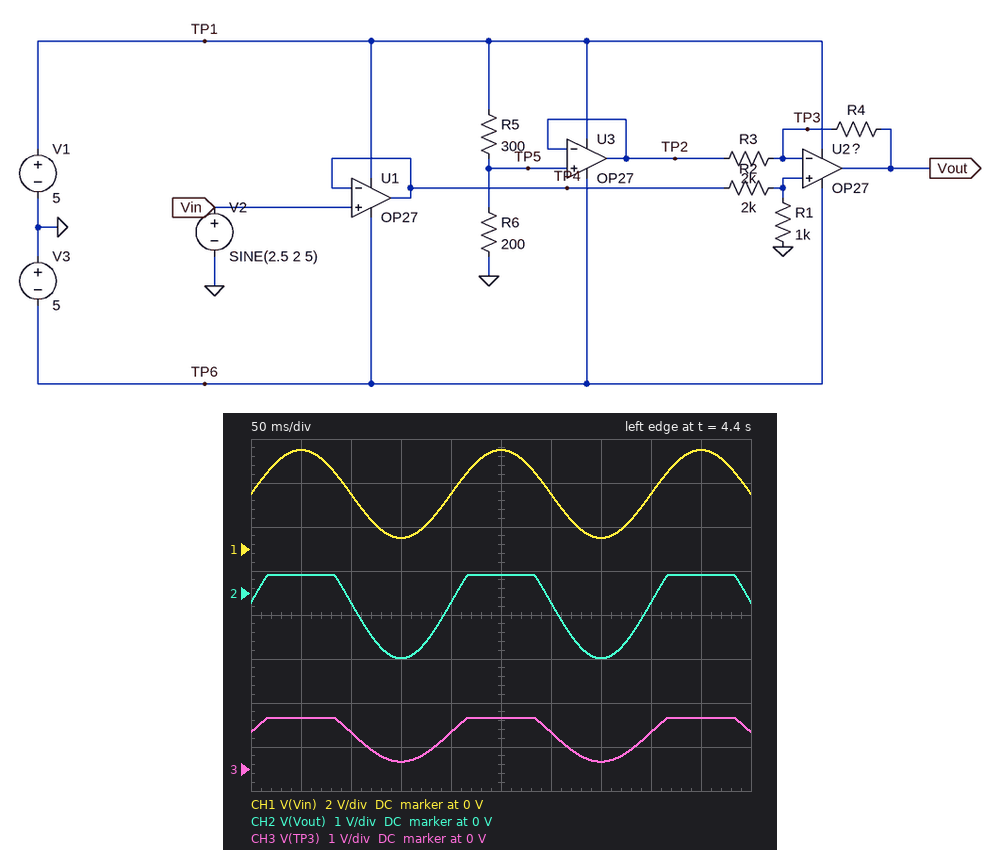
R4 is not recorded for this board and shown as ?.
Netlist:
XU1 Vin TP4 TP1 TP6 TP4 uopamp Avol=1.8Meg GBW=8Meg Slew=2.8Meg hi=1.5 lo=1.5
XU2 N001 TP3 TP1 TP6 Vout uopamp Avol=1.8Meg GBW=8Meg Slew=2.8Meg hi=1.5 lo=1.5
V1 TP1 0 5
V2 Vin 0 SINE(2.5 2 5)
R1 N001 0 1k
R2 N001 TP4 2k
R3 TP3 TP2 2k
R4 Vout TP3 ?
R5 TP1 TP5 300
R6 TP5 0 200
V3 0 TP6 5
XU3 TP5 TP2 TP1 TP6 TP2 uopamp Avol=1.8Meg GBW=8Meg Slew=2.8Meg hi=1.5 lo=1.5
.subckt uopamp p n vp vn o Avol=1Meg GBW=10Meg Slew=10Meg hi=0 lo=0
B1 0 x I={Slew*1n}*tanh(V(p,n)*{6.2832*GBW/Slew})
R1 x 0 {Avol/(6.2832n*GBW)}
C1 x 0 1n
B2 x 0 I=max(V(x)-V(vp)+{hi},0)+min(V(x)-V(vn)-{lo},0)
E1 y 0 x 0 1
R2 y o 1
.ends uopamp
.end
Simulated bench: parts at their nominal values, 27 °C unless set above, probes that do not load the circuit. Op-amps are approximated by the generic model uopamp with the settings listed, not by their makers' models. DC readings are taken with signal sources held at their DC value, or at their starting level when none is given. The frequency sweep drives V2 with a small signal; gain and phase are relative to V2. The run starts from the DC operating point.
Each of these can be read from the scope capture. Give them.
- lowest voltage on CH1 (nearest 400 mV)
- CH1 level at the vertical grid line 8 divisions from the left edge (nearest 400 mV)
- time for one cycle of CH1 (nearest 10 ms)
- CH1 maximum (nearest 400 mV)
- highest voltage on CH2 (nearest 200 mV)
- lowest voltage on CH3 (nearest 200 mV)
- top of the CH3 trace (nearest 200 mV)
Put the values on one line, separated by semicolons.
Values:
400 mV; 2.4 V; 200 ms; 4.4 V; 400 mV; 200 mV; 1.2 V
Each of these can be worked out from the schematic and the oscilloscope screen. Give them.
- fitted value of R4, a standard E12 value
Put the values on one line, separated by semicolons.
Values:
1.8 kΩ
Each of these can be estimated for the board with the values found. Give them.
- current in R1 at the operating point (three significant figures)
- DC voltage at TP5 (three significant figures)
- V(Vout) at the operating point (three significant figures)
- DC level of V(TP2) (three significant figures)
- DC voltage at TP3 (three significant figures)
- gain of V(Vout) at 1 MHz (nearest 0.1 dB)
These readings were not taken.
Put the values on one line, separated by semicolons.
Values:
833 µA; 2.00 V; -217 mV; 2.00 V; 833 mV; -4.3 dB
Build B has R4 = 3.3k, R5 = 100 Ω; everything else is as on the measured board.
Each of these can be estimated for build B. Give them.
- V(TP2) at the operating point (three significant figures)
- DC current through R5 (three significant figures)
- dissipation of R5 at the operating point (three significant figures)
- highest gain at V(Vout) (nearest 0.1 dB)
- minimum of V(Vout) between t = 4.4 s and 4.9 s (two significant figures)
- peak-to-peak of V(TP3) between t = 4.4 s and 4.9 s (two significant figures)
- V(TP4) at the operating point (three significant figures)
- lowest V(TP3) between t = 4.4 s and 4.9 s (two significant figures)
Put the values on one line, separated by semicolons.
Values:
3.33 V; 16.7 mA; 27.8 mW; -1.1 dB; -3.5 V; 410 mV; 2.50 V; 750 mV
